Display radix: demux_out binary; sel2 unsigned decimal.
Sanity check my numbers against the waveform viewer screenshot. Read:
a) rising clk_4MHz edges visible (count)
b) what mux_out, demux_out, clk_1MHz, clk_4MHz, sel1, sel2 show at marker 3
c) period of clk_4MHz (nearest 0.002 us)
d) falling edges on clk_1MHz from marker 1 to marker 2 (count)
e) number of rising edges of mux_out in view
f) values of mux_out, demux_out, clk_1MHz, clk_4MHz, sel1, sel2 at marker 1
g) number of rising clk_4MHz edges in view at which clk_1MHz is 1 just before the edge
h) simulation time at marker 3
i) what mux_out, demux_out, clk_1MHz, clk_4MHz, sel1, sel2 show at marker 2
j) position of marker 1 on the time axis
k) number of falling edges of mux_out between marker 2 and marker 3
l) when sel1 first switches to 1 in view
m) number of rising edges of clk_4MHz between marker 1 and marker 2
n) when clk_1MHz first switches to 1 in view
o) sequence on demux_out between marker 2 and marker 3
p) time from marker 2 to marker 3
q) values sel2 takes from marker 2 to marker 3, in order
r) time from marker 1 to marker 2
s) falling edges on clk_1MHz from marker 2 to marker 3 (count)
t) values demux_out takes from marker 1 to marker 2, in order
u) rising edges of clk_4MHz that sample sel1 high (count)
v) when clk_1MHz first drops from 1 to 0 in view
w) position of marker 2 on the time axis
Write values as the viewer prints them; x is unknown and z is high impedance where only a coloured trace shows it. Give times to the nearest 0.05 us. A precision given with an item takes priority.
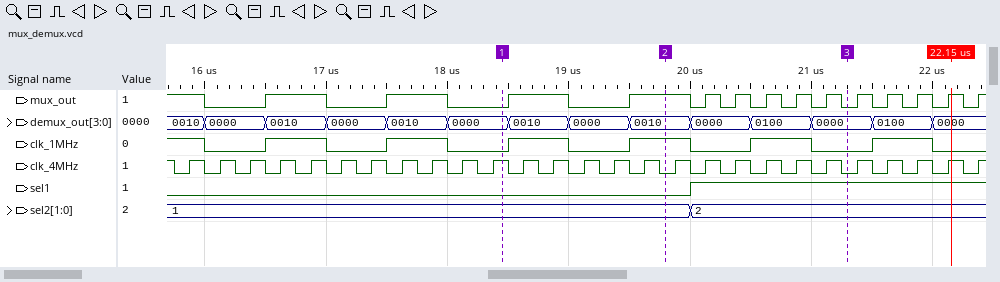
27
mux_out=0, demux_out=0000, clk_1MHz=0, clk_4MHz=0, sel1=1, sel2=2
0.25 us
1
14
mux_out=0, demux_out=0000, clk_1MHz=0, clk_4MHz=1, sel1=0, sel2=1
13
21.3 us
mux_out=1, demux_out=0010, clk_1MHz=1, clk_4MHz=0, sel1=0, sel2=1
18.45 us
6
20 us
5
16.5 us
0010, 0000, 0100, 0000
1.5 us
1, 2
1.35 us
2
0000, 0010, 0000, 0010
10
16 us
19.8 us
